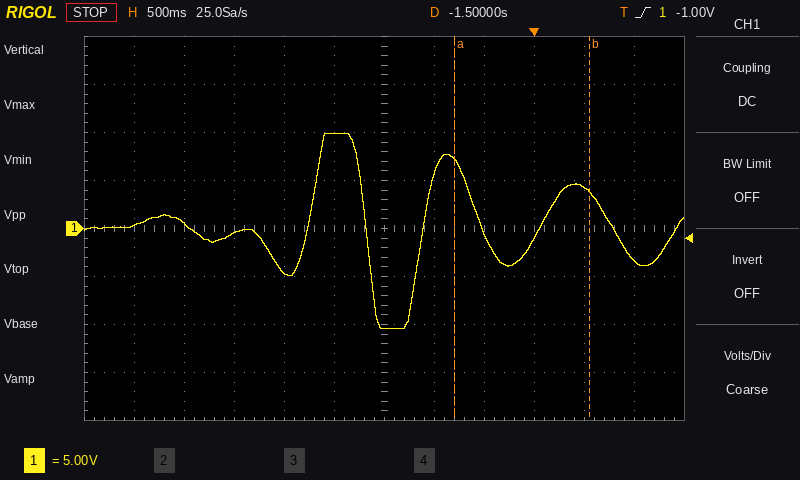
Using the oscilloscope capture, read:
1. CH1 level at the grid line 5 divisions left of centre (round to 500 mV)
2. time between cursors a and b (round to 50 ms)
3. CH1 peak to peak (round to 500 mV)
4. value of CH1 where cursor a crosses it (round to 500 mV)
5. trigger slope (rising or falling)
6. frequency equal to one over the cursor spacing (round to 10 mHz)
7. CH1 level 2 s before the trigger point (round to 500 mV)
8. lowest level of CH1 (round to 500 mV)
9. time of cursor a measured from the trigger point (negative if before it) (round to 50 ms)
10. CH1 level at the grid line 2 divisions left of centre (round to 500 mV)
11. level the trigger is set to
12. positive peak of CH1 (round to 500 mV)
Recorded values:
500 mV
1.35 s
20.5 V
7.0 V
rising
740 mHz
10.0 V
-10.5 V
-800 ms
-4.5 V
-1.00 V
10.0 V
